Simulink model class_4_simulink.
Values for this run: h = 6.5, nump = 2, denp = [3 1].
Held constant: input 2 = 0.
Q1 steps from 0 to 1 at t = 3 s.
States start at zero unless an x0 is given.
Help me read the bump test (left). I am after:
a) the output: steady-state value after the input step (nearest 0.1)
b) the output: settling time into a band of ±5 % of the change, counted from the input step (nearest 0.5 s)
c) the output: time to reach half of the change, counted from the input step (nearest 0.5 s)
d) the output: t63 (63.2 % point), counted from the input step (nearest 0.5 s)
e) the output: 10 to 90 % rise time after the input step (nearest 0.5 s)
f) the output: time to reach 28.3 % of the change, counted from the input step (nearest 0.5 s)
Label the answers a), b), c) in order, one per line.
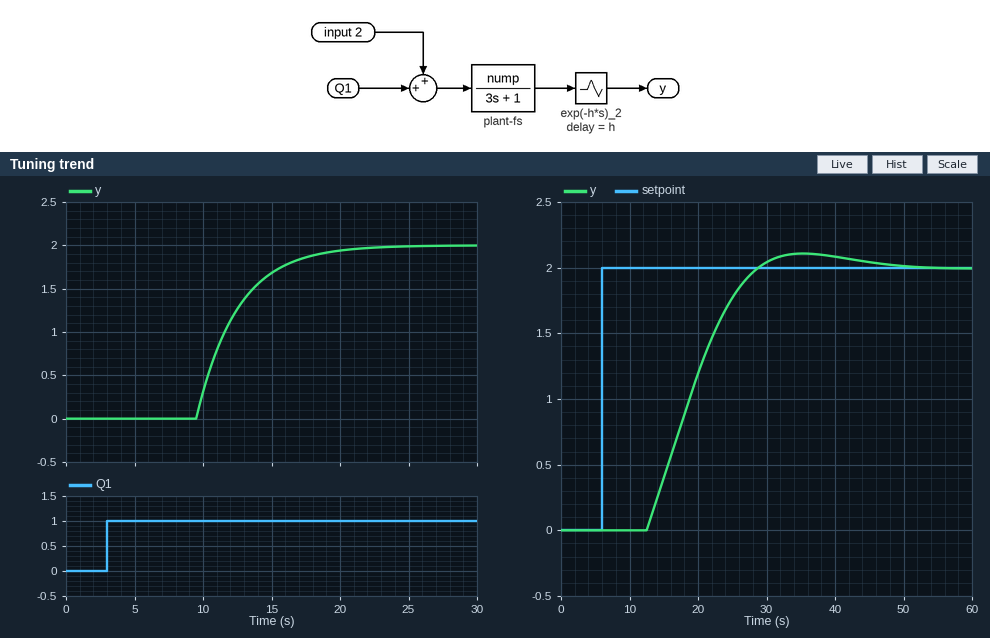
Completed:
a) 2.0
b) 15.5 s
c) 8.5 s
d) 9.5 s
e) 6.5 s
f) 7.5 s
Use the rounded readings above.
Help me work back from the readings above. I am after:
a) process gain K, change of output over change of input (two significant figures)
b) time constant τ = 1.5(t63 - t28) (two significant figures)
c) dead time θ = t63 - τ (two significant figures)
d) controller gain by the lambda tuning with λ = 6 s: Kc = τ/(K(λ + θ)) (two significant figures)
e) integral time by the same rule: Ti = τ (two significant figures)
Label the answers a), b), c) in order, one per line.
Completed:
a) 2.0
b) 3.0 s
c) 6.5 s
d) 0.12
e) 3.0 s
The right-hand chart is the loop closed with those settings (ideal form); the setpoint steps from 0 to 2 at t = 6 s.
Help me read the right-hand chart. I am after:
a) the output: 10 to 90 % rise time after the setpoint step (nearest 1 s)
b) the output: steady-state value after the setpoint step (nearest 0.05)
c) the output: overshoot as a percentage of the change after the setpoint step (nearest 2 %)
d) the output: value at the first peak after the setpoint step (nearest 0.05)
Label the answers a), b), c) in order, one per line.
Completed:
a) 12 s
b) 2.00
c) 6 %
d) 2.10
